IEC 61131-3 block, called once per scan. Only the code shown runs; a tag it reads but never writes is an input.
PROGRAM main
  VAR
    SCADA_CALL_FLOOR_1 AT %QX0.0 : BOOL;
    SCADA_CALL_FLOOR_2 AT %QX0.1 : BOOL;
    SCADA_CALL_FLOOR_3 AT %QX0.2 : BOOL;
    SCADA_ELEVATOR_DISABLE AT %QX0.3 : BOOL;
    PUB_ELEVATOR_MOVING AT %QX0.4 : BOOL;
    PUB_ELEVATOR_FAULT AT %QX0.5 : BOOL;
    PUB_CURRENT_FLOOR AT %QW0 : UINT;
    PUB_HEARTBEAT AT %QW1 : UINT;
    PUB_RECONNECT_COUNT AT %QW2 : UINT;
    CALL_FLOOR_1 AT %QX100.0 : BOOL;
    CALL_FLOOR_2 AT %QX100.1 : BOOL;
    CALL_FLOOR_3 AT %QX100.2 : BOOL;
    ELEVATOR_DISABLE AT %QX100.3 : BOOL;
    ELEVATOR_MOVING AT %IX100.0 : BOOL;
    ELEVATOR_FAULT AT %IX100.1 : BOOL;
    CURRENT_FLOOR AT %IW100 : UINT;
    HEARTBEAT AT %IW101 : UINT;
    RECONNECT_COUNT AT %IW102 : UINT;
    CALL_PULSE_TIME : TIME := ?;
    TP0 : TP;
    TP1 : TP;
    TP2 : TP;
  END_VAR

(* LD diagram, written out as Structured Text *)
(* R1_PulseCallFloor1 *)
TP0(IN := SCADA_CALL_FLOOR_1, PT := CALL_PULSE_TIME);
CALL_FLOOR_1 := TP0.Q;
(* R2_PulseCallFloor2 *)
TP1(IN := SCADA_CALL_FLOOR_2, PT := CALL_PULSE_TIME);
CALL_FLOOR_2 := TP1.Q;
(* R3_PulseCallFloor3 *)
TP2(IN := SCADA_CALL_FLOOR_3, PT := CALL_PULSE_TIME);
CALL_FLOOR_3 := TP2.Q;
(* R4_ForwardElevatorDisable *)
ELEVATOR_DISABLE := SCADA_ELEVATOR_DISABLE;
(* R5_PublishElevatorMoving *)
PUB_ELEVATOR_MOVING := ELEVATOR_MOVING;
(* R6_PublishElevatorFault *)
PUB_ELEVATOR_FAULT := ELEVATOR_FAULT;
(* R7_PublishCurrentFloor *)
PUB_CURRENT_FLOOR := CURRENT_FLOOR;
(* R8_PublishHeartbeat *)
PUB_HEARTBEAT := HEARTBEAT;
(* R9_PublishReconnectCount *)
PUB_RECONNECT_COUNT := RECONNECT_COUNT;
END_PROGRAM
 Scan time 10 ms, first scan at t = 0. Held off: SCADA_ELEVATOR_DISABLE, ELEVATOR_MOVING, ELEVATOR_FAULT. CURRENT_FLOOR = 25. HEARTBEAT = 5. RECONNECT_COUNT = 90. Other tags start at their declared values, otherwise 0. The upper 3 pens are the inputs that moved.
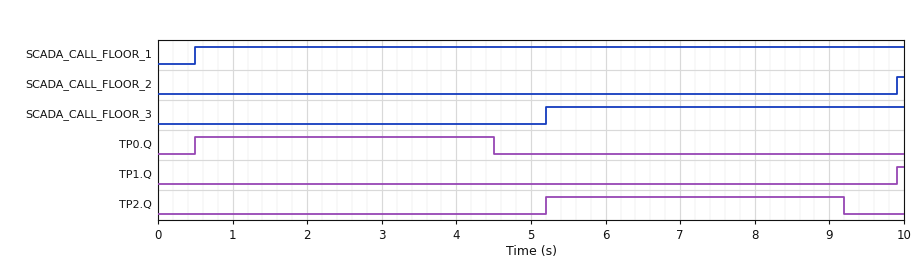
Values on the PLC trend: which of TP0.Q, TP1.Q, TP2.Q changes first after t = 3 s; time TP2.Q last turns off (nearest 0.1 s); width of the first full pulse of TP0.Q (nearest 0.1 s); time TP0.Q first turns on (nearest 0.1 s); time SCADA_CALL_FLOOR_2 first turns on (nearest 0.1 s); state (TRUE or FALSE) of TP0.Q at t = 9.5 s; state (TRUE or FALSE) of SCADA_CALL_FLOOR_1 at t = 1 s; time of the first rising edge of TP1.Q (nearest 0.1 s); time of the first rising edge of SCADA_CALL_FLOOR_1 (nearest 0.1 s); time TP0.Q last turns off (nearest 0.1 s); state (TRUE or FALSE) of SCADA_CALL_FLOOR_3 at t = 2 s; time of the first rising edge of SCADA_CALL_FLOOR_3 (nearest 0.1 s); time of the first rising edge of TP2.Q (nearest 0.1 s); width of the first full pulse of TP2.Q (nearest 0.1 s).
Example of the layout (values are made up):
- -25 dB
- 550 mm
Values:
- TP0.Q
- 9.2 s
- 4.0 s
- 0.5 s
- 9.9 s
- FALSE
- TRUE
- 9.9 s
- 0.5 s
- 4.5 s
- FALSE
- 5.2 s
- 5.2 s
- 4.0 s
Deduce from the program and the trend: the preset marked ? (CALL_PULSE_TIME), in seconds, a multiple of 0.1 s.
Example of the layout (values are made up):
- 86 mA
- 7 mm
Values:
- 4.0 s
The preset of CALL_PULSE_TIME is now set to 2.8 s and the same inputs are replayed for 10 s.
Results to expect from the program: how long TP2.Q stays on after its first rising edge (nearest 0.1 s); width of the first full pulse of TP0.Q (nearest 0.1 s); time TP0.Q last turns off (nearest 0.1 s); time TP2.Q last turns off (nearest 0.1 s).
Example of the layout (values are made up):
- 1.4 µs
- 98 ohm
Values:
- 2.8 s
- 2.8 s
- 3.3 s
- 8.0 s
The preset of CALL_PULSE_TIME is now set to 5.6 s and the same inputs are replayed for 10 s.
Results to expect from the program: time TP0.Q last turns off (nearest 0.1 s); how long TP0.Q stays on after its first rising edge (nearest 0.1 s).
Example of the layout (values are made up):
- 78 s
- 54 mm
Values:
- 6.1 s
- 5.6 s
